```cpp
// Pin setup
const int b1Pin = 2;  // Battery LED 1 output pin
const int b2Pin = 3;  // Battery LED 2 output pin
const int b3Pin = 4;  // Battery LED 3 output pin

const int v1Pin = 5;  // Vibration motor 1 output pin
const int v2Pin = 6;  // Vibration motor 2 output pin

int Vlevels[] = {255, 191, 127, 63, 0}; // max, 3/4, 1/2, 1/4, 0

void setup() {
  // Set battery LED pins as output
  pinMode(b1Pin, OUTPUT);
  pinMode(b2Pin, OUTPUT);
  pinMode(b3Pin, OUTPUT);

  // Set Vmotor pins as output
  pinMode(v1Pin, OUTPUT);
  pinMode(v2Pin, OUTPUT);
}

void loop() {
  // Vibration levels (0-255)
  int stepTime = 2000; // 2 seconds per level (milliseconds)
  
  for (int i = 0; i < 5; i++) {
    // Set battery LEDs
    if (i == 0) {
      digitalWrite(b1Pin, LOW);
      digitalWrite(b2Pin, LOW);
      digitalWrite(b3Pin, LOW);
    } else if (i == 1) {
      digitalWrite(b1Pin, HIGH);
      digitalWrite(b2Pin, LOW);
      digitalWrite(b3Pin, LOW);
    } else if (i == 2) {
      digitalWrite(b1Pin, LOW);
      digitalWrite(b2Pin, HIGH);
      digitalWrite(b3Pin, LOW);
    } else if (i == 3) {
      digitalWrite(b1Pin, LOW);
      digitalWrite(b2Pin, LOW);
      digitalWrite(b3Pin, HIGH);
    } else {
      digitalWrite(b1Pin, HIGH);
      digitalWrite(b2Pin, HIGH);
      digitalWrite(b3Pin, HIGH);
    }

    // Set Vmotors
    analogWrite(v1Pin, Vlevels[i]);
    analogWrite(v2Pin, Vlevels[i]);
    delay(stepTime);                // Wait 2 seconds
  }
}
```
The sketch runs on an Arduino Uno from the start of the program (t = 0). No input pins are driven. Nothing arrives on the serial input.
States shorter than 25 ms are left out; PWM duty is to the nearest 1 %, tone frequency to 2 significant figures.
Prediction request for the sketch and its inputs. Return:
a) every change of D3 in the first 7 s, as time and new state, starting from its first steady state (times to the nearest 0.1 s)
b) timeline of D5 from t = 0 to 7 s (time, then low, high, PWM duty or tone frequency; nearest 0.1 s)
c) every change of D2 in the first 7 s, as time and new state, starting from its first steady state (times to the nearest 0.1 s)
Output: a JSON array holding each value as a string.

["0 s low; 4 s high; 6 s low", "0 s high; 2 s PWM 75 %; 4 s PWM 50 %; 6 s PWM 25 %", "0 s low; 2 s high; 4 s low"]
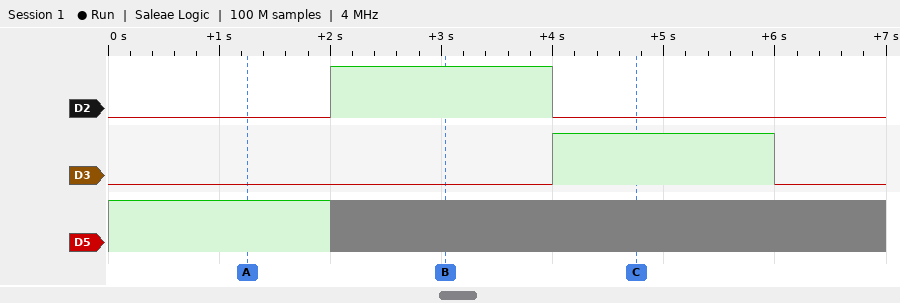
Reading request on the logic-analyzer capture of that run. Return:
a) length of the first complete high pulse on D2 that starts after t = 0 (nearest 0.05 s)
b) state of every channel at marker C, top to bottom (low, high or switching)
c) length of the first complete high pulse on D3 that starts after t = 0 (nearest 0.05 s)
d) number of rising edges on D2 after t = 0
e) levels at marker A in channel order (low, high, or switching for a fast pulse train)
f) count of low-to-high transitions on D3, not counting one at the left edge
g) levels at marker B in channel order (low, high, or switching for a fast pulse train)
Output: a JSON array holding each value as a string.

["2.00 s", "D2 low, D3 high, D5 switching", "2.00 s", "1", "D2 low, D3 low, D5 high", "1", "D2 high, D3 low, D5 switching"]
